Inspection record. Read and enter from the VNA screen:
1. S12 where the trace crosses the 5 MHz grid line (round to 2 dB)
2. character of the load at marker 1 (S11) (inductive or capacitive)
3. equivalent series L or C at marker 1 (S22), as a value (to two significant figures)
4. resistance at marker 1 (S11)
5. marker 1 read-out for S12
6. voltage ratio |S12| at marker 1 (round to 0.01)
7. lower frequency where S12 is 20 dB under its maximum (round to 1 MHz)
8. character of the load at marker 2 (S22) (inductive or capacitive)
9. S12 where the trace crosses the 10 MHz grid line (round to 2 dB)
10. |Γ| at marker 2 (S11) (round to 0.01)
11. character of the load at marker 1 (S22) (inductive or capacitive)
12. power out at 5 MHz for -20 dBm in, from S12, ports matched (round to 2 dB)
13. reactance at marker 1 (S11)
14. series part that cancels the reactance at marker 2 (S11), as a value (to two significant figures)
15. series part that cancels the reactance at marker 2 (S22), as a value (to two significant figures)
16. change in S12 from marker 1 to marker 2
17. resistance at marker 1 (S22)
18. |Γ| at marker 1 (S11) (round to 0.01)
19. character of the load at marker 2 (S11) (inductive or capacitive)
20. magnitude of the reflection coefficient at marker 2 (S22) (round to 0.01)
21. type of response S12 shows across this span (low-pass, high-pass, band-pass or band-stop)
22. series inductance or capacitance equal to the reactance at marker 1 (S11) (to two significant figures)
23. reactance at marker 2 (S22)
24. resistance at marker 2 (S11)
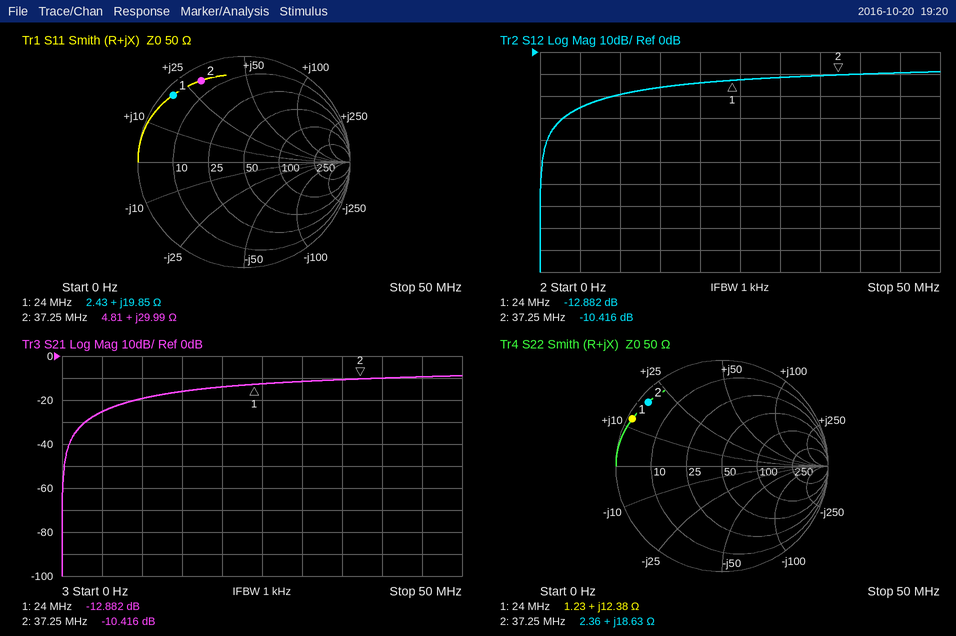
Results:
-26 dB
inductive
82 nH
2.43 Ω
-12.882 dB
0.23
3 MHz
inductive
-20 dB
0.87
inductive
-46 dBm
+19.85 Ω
140 pF
230 pF
2.466 dB
1.23 Ω
0.92
inductive
0.92
high-pass
130 nH
+18.63 Ω
4.81 Ω
